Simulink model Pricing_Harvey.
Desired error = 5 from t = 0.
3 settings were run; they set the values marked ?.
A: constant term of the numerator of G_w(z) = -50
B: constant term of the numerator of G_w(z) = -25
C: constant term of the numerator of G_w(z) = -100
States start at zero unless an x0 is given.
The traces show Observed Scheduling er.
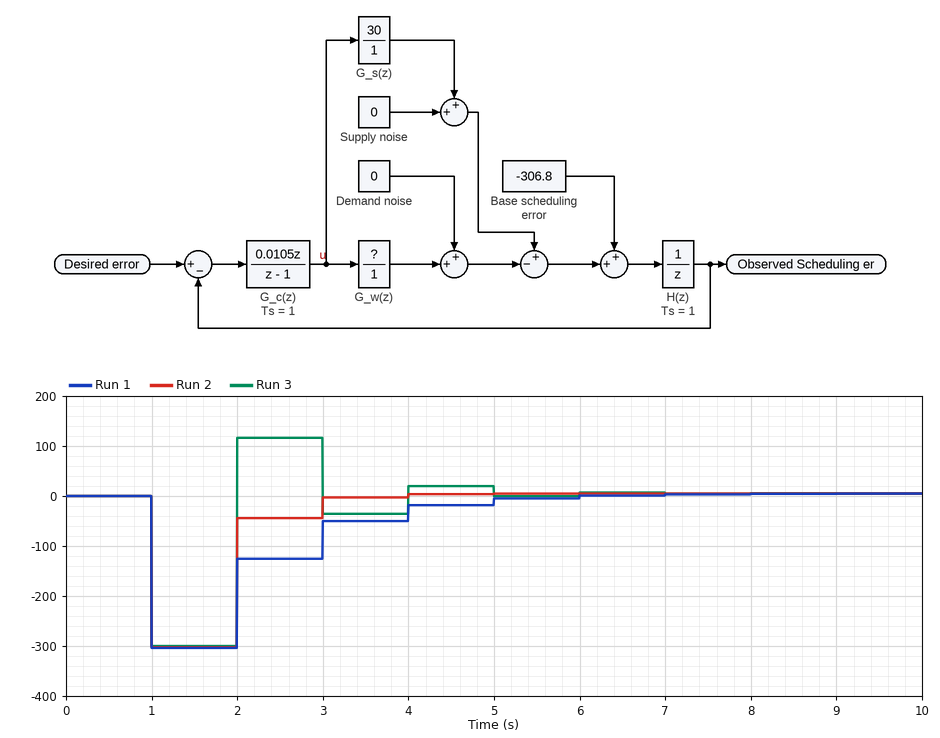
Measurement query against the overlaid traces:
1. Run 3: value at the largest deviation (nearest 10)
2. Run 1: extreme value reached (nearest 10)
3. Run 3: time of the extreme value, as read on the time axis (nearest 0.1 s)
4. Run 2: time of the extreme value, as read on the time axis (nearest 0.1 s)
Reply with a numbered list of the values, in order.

1. -300
2. -300
3. 1.0 s
4. 1.0 s
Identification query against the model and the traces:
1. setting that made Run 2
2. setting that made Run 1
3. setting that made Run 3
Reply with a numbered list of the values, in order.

1. A
2. B
3. C
